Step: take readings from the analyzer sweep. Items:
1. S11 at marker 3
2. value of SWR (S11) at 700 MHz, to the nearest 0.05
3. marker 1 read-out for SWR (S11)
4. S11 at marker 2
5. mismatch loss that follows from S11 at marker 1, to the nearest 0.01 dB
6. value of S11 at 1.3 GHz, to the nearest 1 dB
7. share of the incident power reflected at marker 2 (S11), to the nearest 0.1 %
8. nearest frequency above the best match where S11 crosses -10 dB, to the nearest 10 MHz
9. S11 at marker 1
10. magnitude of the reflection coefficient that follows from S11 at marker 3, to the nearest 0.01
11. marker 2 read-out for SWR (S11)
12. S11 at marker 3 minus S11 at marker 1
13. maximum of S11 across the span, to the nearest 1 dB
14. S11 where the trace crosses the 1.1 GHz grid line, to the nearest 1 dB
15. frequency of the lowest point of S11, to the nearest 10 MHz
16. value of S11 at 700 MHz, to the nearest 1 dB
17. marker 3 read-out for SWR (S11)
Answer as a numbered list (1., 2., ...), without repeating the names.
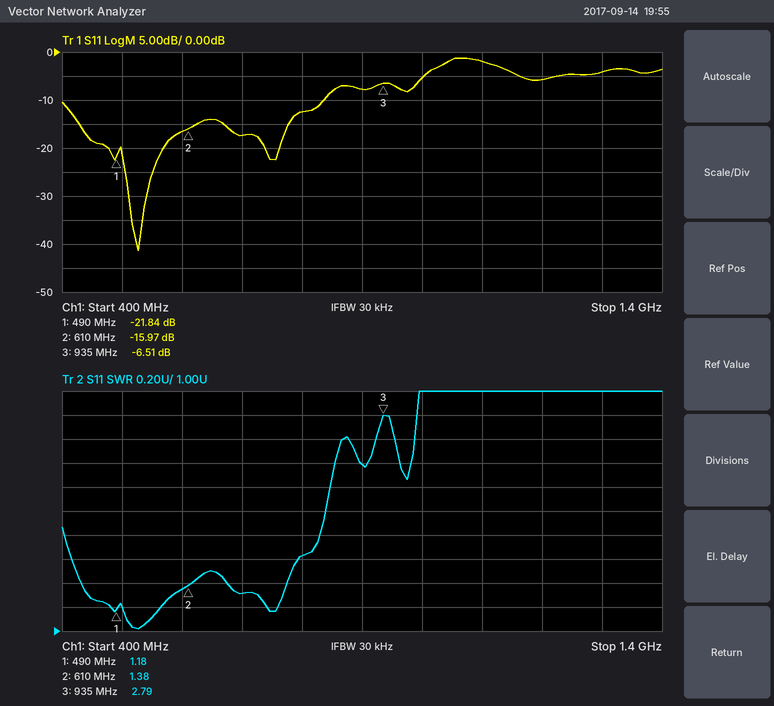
1. -6.51 dB
2. 1.30
3. 1.18
4. -15.97 dB
5. 0.03 dB
6. -4 dB
7. 2.5 %
8. 840 MHz
9. -21.84 dB
10. 0.47
11. 1.38
12. 15.33 dB
13. -1 dB
14. -2 dB
15. 530 MHz
16. -17 dB
17. 2.79
